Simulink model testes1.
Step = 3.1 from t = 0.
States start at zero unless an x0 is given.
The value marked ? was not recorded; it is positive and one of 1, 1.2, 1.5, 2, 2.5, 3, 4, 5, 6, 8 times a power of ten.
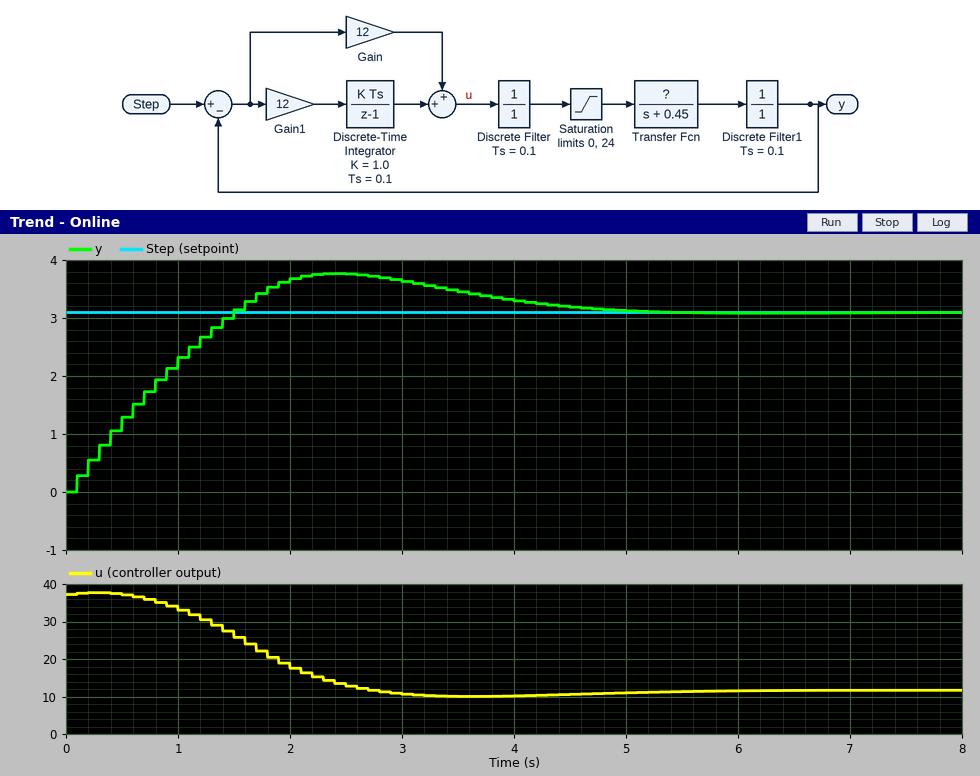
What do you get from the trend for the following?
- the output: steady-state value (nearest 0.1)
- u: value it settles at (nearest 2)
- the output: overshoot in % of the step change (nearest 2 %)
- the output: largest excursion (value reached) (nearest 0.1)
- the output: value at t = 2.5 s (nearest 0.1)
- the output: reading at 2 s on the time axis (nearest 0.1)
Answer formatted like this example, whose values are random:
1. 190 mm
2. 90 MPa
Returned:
1. 3.1
2. 12
3. 22 %
4. 3.8
5. 3.8
6. 3.7
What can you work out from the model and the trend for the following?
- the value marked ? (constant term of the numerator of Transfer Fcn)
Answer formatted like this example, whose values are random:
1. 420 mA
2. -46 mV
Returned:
1. 0.12
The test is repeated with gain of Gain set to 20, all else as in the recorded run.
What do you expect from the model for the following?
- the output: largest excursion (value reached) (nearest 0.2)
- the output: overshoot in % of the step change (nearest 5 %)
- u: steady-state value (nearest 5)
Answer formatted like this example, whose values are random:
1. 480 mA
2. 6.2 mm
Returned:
1. 3.6
2. 15 %
3. 10
